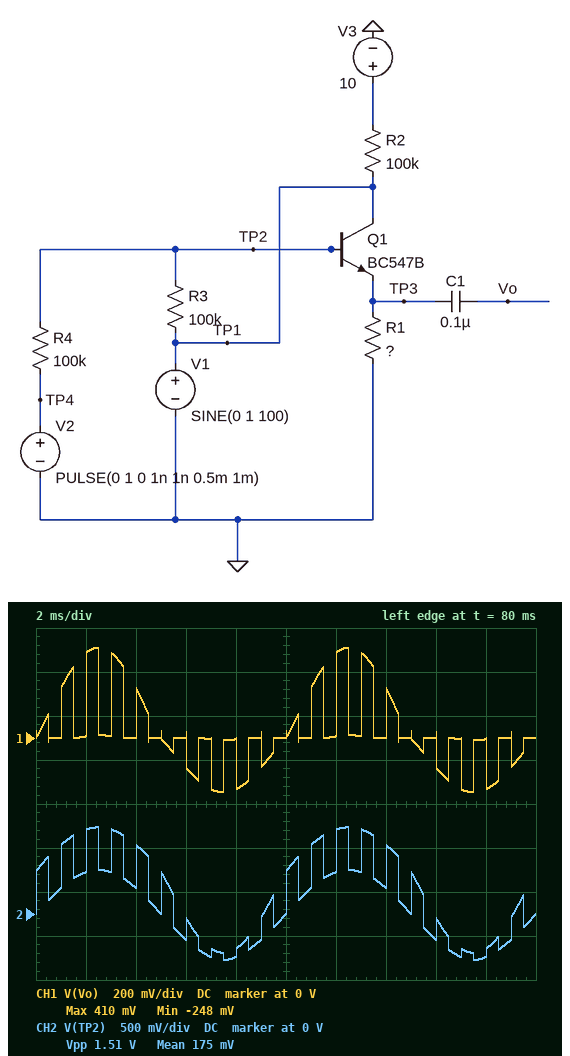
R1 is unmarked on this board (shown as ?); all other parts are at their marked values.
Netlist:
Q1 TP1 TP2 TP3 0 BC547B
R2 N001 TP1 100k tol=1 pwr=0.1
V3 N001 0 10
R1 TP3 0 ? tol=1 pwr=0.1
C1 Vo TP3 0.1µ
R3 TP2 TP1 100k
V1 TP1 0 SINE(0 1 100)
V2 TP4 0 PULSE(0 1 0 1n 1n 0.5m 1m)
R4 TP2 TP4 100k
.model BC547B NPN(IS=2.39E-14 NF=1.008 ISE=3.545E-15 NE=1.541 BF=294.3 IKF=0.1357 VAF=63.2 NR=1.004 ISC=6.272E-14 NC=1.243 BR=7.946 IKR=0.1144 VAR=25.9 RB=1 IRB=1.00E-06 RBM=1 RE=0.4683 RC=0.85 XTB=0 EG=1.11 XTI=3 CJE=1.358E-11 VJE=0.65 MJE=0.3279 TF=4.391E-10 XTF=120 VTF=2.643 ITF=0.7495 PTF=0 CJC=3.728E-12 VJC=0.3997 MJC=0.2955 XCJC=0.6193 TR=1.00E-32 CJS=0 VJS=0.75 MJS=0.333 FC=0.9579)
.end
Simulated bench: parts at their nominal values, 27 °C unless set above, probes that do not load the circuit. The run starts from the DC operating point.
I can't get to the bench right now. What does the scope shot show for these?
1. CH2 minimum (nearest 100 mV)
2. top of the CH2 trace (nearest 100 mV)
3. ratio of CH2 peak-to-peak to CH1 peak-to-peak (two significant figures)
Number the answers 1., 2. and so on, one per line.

1. -500 mV
2. 1.0 V
3. 2.3
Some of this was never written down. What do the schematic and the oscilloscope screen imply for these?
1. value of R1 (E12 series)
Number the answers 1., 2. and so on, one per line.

1. 4.7 kΩ
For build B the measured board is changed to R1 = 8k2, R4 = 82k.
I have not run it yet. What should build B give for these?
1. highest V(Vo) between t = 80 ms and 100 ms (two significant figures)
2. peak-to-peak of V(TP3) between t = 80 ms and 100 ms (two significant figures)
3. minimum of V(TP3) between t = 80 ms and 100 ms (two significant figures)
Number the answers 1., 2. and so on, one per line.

1. 430 mV
2. 1.0 V
3. -580 mV
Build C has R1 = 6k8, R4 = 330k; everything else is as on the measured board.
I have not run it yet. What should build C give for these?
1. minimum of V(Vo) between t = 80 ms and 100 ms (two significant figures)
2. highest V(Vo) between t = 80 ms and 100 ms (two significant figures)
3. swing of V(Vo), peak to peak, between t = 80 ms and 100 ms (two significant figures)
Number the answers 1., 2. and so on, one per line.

1. -13 mV
2. 420 mV
3. 430 mV
